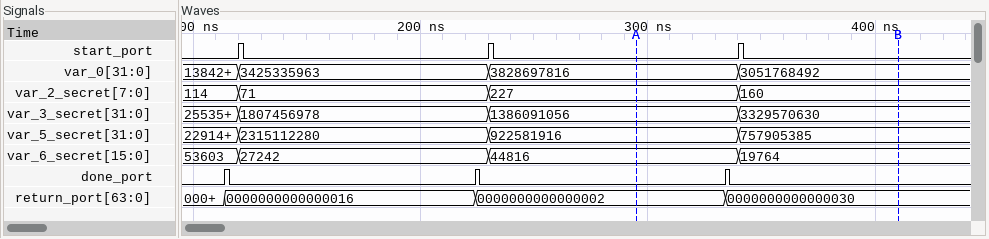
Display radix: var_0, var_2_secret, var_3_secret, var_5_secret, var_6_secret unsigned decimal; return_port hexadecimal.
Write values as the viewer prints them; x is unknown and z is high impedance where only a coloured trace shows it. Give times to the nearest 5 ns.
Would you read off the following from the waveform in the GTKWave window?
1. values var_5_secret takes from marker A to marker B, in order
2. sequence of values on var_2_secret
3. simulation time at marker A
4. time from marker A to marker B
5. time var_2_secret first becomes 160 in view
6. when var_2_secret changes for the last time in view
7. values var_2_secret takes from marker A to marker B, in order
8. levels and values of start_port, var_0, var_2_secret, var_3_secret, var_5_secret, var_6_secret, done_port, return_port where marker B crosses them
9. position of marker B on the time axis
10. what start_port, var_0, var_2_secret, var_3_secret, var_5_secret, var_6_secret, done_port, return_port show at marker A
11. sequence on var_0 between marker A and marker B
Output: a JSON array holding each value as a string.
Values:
["922581916, 757905385", "114, 71, 227, 160", "295 ns", "115 ns", "340 ns", "340 ns", "227, 160", "start_port=0, var_0=3051768492, var_2_secret=160, var_3_secret=3329570630, var_5_secret=757905385, var_6_secret=19764, done_port=0, return_port=0000000000000030", "410 ns", "start_port=0, var_0=3828697816, var_2_secret=227, var_3_secret=1386091056, var_5_secret=922581916, var_6_secret=44816, done_port=0, return_port=0000000000000002", "3828697816, 3051768492"]
